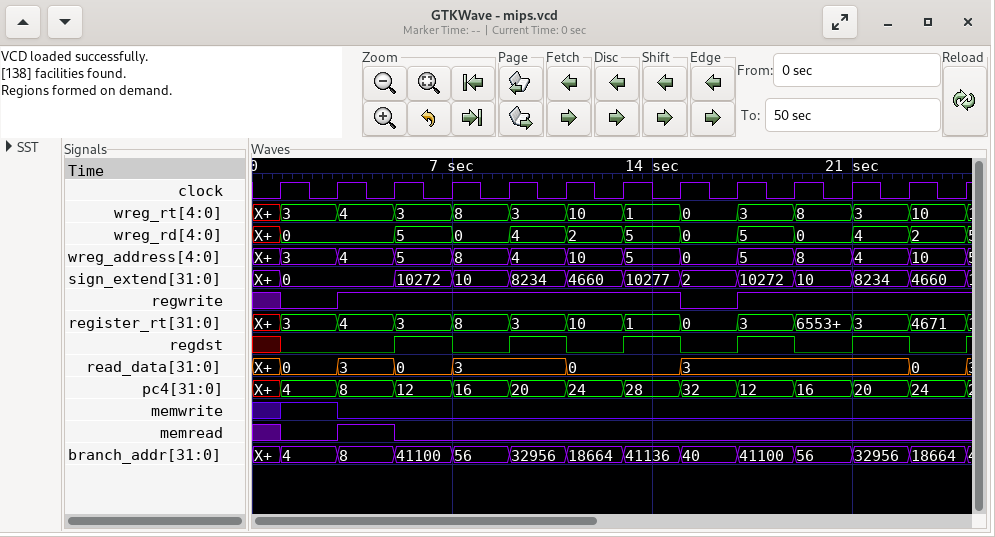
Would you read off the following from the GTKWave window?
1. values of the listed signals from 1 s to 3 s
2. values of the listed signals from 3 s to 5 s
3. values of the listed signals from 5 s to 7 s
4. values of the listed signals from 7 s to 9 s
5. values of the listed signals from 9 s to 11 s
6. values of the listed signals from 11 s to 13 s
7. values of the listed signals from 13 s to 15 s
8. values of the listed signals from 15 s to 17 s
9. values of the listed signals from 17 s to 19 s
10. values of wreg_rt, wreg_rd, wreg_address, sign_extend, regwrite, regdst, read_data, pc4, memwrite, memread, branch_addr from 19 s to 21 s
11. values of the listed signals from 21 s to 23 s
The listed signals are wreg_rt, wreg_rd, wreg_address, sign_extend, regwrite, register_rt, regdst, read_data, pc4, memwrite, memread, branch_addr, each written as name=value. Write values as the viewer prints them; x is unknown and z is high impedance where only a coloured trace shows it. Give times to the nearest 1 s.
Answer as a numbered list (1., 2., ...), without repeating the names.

1. wreg_rt=3, wreg_rd=0, wreg_address=3, sign_extend=0, regwrite=0, register_rt=3, regdst=0, read_data=0, pc4=4, memwrite=1, memread=0, branch_addr=4
2. wreg_rt=4, wreg_rd=0, wreg_address=4, sign_extend=0, regwrite=1, register_rt=4, regdst=0, read_data=3, pc4=8, memwrite=0, memread=1, branch_addr=8
3. wreg_rt=3, wreg_rd=5, wreg_address=5, sign_extend=10272, regwrite=1, register_rt=3, regdst=1, read_data=0, pc4=12, memwrite=0, memread=0, branch_addr=41100
4. wreg_rt=8, wreg_rd=0, wreg_address=8, sign_extend=10, regwrite=1, register_rt=8, regdst=0, read_data=3, pc4=16, memwrite=0, memread=0, branch_addr=56
5. wreg_rt=3, wreg_rd=4, wreg_address=4, sign_extend=8234, regwrite=1, register_rt=3, regdst=1, read_data=3, pc4=20, memwrite=0, memread=0, branch_addr=32956
6. wreg_rt=10, wreg_rd=2, wreg_address=10, sign_extend=4660, regwrite=1, register_rt=10, regdst=0, read_data=0, pc4=24, memwrite=0, memread=0, branch_addr=18664
7. wreg_rt=1, wreg_rd=5, wreg_address=5, sign_extend=10277, regwrite=1, register_rt=1, regdst=1, read_data=0, pc4=28, memwrite=0, memread=0, branch_addr=41136
8. wreg_rt=0, wreg_rd=0, wreg_address=0, sign_extend=2, regwrite=0, register_rt=0, regdst=0, read_data=3, pc4=32, memwrite=0, memread=0, branch_addr=40
9. wreg_rt=3, wreg_rd=5, wreg_address=5, sign_extend=10272, regwrite=1, register_rt=3, regdst=1, read_data=3, pc4=12, memwrite=0, memread=0, branch_addr=41100
10. wreg_rt=8, wreg_rd=0, wreg_address=8, sign_extend=10, regwrite=1, regdst=0, read_data=3, pc4=16, memwrite=0, memread=0, branch_addr=56
11. wreg_rt=3, wreg_rd=4, wreg_address=4, sign_extend=8234, regwrite=1, register_rt=3, regdst=1, read_data=3, pc4=20, memwrite=0, memread=0, branch_addr=32956
